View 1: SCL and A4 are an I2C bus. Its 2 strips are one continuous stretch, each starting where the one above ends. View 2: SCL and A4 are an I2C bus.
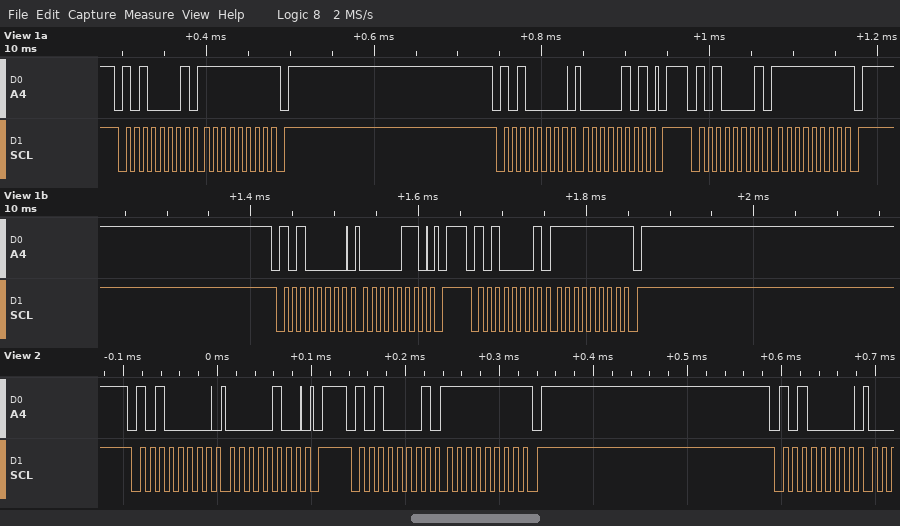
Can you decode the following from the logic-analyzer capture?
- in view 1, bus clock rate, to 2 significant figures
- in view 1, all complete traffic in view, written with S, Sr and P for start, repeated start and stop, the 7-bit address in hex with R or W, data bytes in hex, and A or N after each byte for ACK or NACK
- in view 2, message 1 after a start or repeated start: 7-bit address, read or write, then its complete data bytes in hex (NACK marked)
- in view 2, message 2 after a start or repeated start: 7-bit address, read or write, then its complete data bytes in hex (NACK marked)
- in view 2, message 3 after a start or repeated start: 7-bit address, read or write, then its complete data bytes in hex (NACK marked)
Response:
100 kHz
S 50R A FF N P S 50W A 05 A P S 50R A FF N P S 50W A 06 A P S 50R A FF N P
0x50 write: 04
0x50 read: FF NACK
0x50 write
